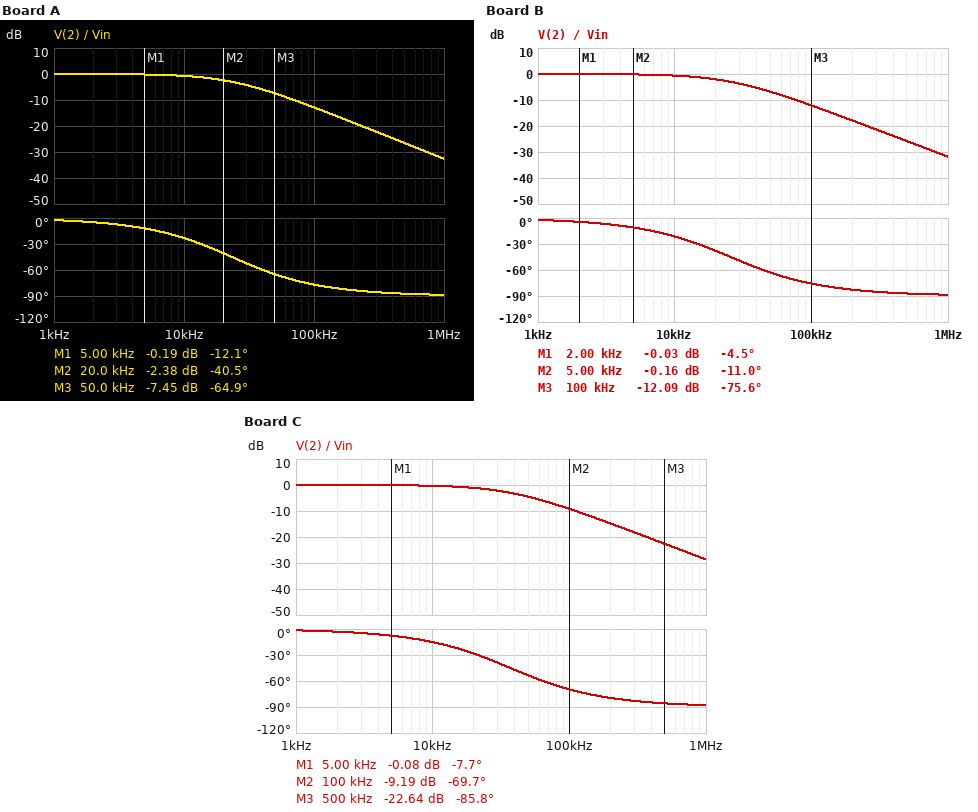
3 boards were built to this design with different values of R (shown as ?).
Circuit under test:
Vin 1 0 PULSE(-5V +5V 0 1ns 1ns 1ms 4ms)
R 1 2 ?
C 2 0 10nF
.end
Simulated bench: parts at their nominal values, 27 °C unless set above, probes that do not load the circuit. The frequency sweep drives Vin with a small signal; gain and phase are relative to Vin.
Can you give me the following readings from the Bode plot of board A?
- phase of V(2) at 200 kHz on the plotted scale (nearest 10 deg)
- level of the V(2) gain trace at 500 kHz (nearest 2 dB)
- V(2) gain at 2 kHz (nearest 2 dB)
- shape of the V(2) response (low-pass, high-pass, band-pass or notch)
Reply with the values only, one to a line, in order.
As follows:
-80 deg
-26 dB
0 dB
low-pass
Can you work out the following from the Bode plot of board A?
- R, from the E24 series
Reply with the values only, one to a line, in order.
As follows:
680 Ω
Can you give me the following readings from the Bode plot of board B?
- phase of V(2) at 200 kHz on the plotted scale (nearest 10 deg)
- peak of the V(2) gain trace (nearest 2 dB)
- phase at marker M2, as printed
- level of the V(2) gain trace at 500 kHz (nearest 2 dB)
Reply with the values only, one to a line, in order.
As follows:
-80 deg
0 dB
-11.0 deg
-26 dB
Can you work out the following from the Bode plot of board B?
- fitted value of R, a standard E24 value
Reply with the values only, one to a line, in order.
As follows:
620 Ω
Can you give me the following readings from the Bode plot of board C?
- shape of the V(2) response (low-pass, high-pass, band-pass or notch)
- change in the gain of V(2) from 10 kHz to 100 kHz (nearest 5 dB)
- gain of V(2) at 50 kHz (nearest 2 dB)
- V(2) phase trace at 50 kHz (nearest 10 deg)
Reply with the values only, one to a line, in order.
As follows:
low-pass
-10 dB
-4 dB
-50 deg
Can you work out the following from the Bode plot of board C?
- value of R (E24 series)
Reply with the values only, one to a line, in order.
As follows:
430 Ω
